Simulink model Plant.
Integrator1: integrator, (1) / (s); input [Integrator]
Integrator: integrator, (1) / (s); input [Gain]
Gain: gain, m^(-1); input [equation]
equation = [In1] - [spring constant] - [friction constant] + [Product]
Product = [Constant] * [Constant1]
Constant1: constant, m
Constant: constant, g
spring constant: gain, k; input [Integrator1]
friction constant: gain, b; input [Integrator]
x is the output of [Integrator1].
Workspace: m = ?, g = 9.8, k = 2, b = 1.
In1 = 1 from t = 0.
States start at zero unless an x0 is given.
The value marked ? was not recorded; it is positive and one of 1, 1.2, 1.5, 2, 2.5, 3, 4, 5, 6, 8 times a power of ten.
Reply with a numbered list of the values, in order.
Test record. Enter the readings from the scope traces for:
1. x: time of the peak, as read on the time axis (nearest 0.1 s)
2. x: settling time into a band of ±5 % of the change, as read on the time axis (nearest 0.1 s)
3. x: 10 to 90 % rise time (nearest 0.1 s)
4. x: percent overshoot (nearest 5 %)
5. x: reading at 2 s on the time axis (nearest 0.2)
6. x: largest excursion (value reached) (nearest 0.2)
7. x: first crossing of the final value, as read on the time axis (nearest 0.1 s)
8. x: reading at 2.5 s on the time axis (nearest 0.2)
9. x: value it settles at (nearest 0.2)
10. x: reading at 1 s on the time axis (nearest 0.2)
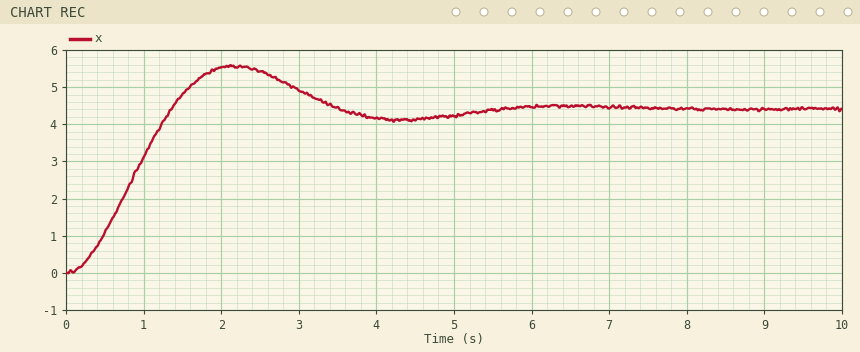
1. 2.2 s
2. 4.8 s
3. 0.9 s
4. 25 %
5. 5.6
6. 5.6
7. 1.4 s
8. 5.4
9. 4.4
10. 3.2
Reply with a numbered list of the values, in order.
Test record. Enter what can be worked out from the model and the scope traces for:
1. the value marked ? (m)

1. 0.8
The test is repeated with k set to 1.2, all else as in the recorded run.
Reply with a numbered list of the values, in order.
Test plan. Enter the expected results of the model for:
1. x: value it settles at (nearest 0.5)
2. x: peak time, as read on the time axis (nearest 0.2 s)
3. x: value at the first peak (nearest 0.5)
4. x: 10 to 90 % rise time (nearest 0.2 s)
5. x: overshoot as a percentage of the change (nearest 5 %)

1. 7.5
2. 3.0 s
3. 8.5
4. 1.4 s
5. 15 %
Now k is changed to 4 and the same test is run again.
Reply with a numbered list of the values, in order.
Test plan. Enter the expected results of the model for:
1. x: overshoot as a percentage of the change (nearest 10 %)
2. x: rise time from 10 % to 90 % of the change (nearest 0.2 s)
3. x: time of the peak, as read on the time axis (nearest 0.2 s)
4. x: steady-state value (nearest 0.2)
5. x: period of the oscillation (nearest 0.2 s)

1. 40 %
2. 0.6 s
3. 1.4 s
4. 2.2
5. 3.0 s
